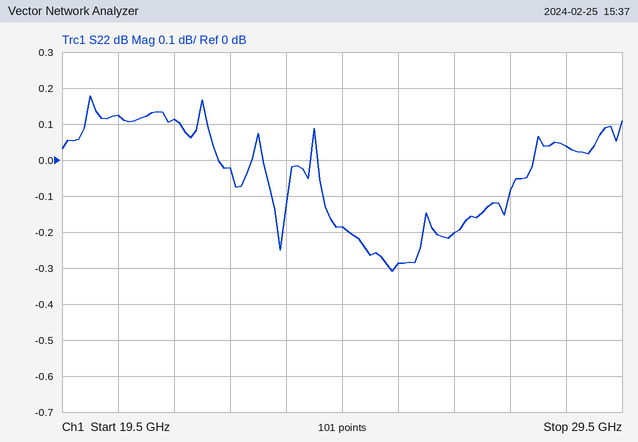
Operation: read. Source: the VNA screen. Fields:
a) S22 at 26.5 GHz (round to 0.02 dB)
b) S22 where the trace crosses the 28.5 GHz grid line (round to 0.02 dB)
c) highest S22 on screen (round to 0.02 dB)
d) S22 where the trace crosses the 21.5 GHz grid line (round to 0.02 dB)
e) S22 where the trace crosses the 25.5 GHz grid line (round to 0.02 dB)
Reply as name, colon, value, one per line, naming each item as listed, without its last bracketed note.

S22 at 26.5 GHz: -0.20 dB
S22 where the trace crosses the 28.5 GHz grid line: 0.04 dB
highest S22 on screen: 0.18 dB
S22 where the trace crosses the 21.5 GHz grid line: 0.12 dB
S22 where the trace crosses the 25.5 GHz grid line: -0.28 dB
